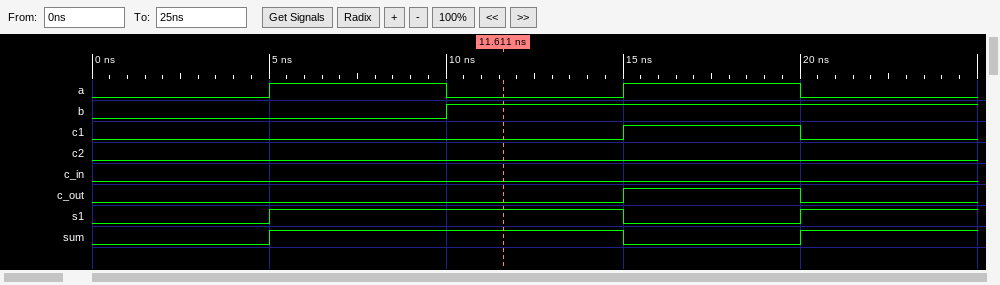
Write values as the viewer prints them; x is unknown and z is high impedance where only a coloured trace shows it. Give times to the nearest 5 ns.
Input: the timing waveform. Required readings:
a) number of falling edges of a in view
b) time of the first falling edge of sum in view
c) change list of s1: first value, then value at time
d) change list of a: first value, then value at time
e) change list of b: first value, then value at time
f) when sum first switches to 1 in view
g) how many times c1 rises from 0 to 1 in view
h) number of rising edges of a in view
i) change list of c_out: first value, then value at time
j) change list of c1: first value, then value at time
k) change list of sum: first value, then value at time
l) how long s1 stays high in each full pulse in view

2
15 ns
0, 1 at 5 ns, 0 at 15 ns, 1 at 20 ns
0, 1 at 5 ns, 0 at 10 ns, 1 at 15 ns, 0 at 20 ns
0, 1 at 10 ns
5 ns
1
2
0, 1 at 15 ns, 0 at 20 ns
0, 1 at 15 ns, 0 at 20 ns
0, 1 at 5 ns, 0 at 15 ns, 1 at 20 ns
10 ns
